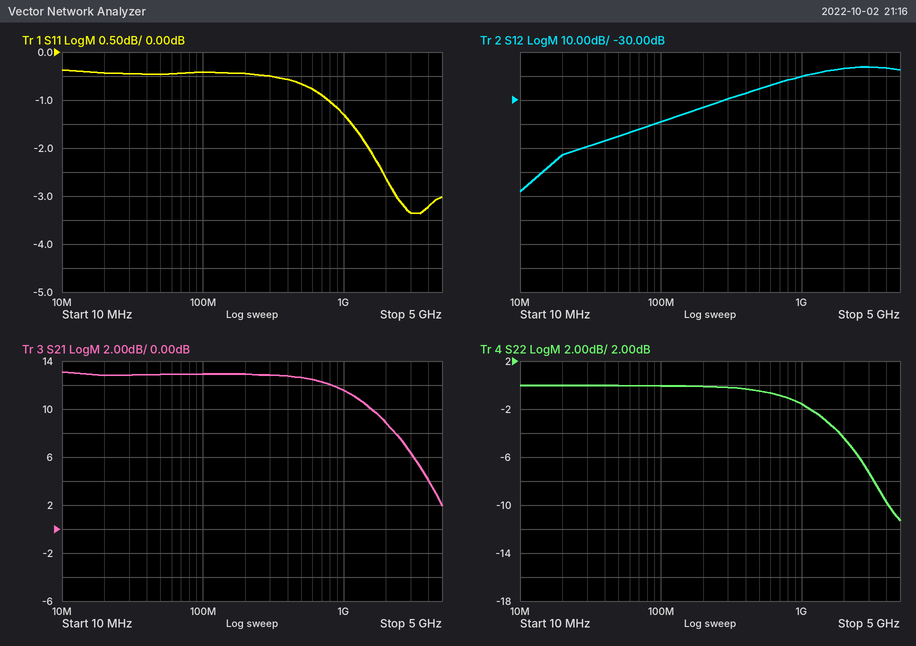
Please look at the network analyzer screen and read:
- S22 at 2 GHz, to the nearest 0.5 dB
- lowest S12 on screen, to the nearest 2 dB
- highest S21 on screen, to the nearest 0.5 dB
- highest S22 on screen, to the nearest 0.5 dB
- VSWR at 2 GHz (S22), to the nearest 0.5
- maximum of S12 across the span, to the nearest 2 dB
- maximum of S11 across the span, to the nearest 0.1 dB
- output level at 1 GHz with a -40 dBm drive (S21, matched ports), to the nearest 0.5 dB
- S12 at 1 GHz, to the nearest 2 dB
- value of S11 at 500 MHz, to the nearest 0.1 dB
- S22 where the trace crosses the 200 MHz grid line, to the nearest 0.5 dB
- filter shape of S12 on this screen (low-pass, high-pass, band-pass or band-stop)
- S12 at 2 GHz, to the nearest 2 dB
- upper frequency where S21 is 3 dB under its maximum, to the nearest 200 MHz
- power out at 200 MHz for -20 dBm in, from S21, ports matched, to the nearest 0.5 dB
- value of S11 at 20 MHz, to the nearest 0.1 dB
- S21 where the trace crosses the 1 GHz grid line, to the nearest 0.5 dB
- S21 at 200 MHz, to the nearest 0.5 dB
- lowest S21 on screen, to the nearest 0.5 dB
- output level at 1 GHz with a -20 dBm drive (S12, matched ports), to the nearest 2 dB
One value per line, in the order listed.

-4.5 dB
-68 dB
13.0 dB
0.0 dB
4.0
-16 dB
-0.4 dB
-28.5 dBm
-20 dB
-0.7 dB
0.0 dB
high-pass
-16 dB
1.6 GHz
-7.0 dBm
-0.4 dB
11.5 dB
13.0 dB
2.0 dB
-40 dBm
